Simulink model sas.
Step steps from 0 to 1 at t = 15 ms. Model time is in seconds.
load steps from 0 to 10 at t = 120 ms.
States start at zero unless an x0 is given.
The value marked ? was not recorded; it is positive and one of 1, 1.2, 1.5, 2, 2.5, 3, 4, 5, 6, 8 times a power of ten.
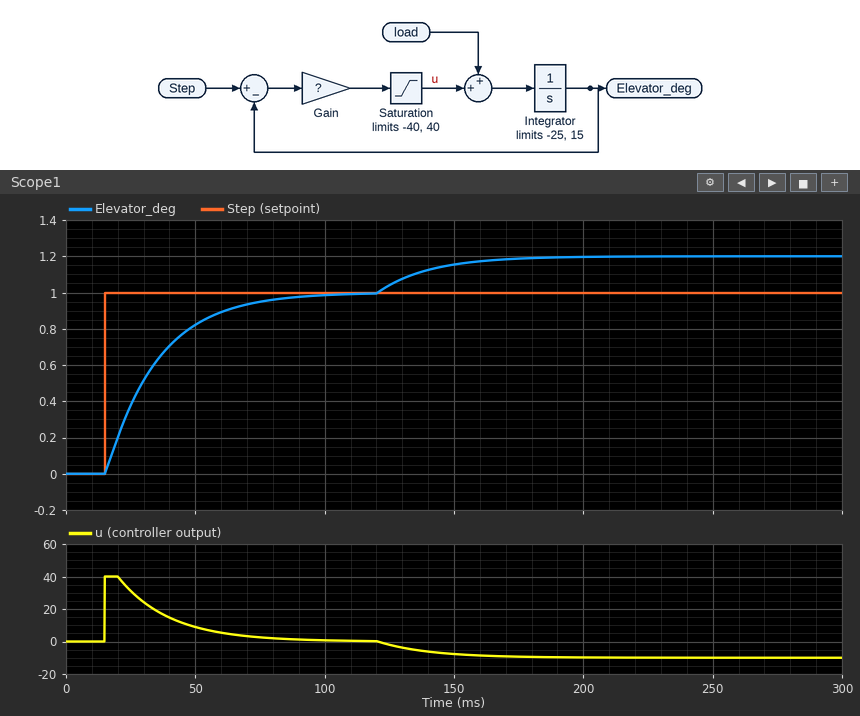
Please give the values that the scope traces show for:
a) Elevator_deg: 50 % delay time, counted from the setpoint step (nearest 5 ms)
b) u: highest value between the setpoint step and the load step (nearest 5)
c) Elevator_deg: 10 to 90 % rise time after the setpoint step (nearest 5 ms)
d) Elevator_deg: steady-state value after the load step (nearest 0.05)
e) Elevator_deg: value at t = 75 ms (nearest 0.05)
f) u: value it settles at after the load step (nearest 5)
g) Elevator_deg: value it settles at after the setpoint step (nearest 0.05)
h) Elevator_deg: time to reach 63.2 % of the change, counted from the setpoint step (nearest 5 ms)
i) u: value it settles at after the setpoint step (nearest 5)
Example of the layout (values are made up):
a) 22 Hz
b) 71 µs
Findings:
a) 15 ms
b) 40
c) 45 ms
d) 1.20
e) 0.95
f) -10
g) 1.00
h) 20 ms
i) 0
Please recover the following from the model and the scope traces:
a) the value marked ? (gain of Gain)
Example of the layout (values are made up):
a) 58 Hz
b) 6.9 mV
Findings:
a) 50
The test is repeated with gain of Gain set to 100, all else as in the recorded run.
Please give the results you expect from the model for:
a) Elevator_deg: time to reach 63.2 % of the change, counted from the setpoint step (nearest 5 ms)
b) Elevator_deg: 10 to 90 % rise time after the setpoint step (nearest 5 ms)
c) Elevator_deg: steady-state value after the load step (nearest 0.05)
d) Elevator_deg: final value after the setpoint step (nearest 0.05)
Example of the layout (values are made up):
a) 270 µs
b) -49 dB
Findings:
a) 15 ms
b) 25 ms
c) 1.10
d) 1.00
